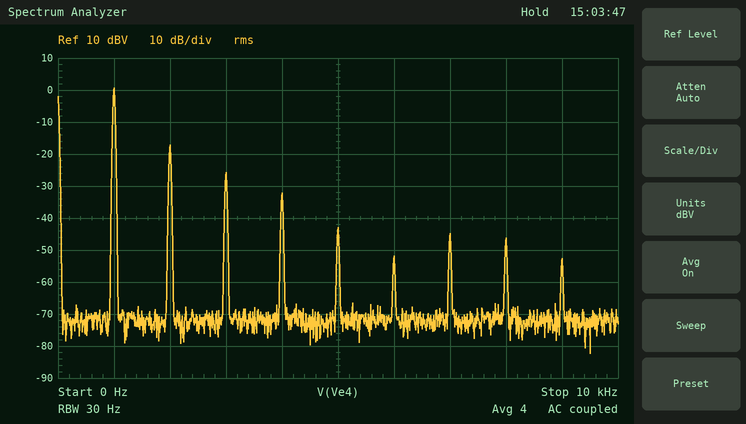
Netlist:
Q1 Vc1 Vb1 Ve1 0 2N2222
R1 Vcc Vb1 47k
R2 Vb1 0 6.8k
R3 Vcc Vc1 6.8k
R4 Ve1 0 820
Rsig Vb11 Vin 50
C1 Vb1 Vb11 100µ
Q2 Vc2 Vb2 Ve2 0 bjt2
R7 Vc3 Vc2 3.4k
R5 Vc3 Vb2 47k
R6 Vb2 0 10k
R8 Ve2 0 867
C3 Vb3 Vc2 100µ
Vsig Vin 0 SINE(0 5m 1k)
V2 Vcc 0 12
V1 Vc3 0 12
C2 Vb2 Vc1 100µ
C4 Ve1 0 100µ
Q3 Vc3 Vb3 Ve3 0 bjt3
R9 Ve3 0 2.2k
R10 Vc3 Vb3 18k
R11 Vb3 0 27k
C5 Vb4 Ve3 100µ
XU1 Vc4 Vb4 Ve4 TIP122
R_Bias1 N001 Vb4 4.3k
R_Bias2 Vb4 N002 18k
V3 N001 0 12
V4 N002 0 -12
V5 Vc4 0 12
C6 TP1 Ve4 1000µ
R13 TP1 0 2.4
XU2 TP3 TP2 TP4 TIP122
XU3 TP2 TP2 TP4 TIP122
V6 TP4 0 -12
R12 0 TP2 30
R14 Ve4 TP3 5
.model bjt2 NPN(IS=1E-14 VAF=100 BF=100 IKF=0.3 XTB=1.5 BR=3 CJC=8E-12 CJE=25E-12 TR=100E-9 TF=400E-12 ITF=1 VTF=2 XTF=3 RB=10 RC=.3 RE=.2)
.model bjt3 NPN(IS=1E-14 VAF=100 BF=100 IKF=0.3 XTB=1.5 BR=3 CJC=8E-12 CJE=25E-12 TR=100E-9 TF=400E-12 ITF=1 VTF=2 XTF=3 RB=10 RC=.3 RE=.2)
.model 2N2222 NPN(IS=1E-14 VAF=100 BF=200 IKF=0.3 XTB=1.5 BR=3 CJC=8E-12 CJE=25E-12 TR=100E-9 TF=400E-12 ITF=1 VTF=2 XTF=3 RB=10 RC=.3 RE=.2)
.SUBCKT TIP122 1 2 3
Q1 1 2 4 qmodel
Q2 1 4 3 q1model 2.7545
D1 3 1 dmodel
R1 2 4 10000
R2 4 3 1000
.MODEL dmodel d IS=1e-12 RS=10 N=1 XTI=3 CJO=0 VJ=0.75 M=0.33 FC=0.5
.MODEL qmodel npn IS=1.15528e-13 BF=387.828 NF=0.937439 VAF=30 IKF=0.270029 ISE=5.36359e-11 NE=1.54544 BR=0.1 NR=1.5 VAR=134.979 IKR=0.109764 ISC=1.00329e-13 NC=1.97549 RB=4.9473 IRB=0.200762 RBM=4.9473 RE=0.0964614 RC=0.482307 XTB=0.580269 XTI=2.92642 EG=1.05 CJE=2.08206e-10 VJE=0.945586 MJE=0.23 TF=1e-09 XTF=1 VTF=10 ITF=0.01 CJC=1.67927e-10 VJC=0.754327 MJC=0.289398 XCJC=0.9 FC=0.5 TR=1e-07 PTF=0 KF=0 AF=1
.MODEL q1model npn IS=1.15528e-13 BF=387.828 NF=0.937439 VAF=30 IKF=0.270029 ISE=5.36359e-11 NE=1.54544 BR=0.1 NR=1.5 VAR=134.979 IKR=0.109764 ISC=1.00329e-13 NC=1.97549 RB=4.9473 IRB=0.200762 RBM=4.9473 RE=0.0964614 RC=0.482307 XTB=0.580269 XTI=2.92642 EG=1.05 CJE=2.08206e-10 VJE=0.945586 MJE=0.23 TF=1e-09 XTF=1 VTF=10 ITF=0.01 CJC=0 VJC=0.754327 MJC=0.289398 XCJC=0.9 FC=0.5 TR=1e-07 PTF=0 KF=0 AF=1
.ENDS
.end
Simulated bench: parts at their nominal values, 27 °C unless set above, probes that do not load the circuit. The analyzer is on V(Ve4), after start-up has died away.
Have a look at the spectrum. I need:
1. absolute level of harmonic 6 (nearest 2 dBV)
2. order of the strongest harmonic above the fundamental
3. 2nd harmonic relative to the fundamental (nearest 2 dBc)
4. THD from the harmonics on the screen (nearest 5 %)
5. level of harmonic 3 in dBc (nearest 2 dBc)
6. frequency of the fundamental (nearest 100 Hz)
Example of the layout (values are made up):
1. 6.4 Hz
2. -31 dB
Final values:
1. -52 dBV
2. 2
3. -18 dBc
4. 15 %
5. -26 dBc
6. 1.0 kHz
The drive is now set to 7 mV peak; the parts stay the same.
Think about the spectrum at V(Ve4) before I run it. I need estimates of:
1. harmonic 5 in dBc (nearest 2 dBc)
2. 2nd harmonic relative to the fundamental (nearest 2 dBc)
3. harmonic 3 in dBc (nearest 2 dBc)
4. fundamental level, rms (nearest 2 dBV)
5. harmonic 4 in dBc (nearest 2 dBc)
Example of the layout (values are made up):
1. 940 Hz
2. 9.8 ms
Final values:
1. -32 dBc
2. -12 dBc
3. -24 dBc
4. 2 dBV
5. -36 dBc
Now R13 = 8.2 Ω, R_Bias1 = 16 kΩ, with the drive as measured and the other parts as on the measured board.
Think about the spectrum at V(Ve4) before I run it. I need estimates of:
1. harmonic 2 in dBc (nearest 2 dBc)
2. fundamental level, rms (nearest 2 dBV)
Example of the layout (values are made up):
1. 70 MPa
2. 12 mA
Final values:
1. -28 dBc
2. 2 dBV
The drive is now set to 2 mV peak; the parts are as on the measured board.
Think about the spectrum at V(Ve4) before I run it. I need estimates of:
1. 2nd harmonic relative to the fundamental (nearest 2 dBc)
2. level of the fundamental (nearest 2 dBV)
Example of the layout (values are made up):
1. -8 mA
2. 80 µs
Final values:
1. -34 dBc
2. -6 dBV
